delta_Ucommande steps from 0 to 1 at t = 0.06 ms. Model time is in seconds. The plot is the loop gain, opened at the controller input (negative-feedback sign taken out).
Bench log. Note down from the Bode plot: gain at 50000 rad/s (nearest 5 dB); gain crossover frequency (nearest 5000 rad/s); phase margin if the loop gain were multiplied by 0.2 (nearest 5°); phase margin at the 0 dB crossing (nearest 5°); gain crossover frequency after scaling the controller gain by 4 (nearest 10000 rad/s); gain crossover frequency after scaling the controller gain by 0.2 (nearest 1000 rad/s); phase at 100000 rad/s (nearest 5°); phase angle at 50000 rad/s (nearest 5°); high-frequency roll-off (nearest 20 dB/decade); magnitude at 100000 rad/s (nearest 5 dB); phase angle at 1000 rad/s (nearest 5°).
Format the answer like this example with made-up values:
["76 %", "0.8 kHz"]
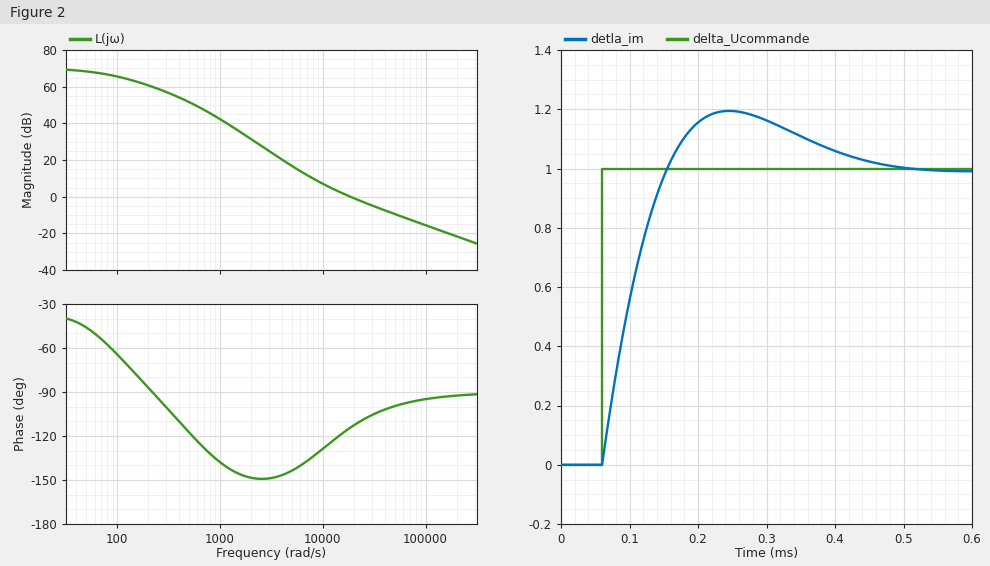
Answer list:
["-10 dB", "20000 rad/s", "40°", "65°", "70000 rad/s", "6000 rad/s", "-95°", "-100°", "-20 dB/decade", "-15 dB", "-140°"]
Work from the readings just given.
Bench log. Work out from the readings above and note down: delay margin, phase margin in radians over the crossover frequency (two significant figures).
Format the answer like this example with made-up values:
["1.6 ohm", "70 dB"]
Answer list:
["0.000057 s"]
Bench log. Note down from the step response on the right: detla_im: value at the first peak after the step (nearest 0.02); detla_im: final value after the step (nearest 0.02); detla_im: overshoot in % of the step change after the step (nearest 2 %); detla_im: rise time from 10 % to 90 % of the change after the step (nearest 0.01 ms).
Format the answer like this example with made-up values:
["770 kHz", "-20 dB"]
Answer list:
["1.20", "1.00", "20 %", "0.07 ms"]
